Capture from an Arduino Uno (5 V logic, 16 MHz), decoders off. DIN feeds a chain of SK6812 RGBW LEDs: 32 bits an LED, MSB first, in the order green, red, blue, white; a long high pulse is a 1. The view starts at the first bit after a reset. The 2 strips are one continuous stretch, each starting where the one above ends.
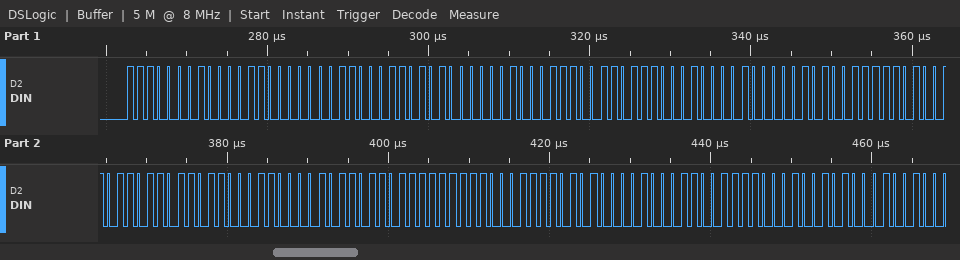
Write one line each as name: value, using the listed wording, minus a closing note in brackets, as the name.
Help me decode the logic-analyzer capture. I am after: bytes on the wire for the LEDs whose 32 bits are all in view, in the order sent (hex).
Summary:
bytes on the wire for the LEDs whose 32 bits are all in view, in the order sent: E1 0C 06 35 02 39 B8 84 14 FA 5B 6C 61 6D FF 1E A1 19 E2 51
